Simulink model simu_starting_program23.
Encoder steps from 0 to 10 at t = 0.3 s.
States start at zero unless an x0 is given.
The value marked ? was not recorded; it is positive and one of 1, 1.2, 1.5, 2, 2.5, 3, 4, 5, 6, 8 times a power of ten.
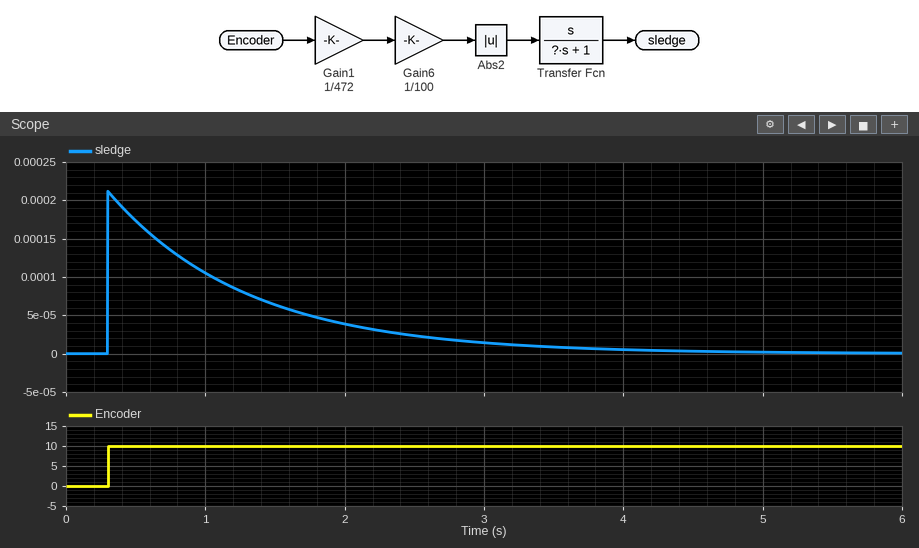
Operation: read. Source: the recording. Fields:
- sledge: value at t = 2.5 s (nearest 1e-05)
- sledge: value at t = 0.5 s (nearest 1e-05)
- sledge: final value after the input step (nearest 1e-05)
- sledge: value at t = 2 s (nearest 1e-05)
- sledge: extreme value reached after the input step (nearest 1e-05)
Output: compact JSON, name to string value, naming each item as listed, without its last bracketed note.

{"sledge: value at t = 2.5 s": "0.00002", "sledge: value at t = 0.5 s": "0.00017", "sledge: final value after the input step": "0.00000", "sledge: value at t = 2 s": "0.00004", "sledge: extreme value reached after the input step": "0.00021"}
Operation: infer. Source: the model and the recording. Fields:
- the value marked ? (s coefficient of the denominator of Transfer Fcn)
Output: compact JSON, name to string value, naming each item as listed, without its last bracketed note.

{"the value marked ?": "1"}
